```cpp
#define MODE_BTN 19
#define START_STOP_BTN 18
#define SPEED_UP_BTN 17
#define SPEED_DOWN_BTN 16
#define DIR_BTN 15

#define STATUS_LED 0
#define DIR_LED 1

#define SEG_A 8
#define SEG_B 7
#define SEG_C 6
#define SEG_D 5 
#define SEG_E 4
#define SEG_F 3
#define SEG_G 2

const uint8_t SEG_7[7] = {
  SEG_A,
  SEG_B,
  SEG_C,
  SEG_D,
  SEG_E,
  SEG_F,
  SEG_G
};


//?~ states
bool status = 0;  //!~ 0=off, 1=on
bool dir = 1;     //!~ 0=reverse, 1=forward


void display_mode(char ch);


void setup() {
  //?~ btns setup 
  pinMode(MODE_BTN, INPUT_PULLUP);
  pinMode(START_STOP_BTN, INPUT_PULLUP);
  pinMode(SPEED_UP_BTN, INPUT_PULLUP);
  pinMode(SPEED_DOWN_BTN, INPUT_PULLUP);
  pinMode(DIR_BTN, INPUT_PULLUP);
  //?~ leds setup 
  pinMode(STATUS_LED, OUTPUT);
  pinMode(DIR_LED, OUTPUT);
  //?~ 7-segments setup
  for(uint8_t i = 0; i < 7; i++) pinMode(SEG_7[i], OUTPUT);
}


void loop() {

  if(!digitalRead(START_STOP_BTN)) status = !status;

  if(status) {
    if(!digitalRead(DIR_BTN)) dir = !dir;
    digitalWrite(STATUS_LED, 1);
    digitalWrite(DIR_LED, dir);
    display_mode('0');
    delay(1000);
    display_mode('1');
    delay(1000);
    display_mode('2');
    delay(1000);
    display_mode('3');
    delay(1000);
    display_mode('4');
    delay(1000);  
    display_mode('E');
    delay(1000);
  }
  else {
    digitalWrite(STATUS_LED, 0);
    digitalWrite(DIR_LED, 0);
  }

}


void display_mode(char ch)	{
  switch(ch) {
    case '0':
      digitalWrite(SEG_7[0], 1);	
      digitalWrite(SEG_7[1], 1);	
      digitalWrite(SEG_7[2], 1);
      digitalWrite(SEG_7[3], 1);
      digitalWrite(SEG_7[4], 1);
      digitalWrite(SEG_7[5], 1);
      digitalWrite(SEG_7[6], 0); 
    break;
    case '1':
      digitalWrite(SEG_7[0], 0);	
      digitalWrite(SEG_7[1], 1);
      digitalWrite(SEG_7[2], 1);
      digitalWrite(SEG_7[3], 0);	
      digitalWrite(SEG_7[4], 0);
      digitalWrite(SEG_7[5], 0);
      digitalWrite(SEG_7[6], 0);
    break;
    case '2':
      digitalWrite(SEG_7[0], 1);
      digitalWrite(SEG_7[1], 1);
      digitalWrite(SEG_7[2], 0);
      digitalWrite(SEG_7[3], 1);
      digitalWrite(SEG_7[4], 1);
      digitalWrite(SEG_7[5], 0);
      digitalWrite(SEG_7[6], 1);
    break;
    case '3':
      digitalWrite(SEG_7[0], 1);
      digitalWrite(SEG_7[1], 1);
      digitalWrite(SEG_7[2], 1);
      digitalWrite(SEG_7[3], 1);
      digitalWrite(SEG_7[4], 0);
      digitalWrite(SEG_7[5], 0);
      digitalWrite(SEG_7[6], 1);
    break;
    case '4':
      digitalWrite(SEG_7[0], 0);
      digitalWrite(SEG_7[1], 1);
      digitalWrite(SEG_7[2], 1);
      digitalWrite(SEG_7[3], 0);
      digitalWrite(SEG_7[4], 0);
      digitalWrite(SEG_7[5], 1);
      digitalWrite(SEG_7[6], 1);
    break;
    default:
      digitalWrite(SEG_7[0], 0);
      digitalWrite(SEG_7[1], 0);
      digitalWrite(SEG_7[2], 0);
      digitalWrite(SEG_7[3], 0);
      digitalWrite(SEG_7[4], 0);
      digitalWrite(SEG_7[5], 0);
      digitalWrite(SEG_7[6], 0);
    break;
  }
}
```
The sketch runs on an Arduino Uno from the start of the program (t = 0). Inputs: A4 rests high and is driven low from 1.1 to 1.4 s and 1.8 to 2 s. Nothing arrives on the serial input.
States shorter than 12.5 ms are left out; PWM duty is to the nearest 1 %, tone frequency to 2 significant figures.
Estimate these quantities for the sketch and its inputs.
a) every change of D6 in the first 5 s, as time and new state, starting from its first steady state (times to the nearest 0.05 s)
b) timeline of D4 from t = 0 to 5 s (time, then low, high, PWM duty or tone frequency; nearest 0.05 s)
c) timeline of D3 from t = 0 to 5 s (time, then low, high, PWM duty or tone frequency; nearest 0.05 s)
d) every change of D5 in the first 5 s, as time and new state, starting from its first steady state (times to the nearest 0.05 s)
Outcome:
0 s low; 1.1 s high; 3.1 s low; 4.1 s high
0 s low; 1.1 s high; 2.1 s low; 3.1 s high; 4.1 s low
0 s low; 1.1 s high; 2.1 s low
0 s low; 1.1 s high; 2.1 s low; 3.1 s high
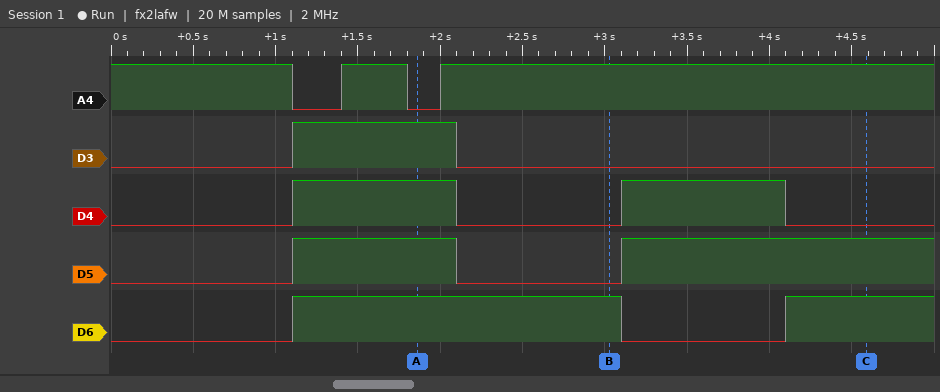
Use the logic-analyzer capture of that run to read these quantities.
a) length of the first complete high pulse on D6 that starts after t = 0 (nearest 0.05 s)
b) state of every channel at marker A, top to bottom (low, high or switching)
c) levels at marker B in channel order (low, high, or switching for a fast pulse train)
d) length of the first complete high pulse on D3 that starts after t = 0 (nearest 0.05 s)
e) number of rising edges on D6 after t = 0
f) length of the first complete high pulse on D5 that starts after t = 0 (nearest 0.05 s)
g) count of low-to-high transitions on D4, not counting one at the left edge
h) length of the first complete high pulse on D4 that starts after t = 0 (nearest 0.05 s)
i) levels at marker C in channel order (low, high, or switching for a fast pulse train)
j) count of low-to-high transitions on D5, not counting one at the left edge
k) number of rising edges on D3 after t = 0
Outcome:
2.00 s
A4 low, D3 high, D4 high, D5 high, D6 high
A4 high, D3 low, D4 low, D5 low, D6 high
1.00 s
2
1.00 s
2
1.00 s
A4 high, D3 low, D4 low, D5 high, D6 high
2
1
